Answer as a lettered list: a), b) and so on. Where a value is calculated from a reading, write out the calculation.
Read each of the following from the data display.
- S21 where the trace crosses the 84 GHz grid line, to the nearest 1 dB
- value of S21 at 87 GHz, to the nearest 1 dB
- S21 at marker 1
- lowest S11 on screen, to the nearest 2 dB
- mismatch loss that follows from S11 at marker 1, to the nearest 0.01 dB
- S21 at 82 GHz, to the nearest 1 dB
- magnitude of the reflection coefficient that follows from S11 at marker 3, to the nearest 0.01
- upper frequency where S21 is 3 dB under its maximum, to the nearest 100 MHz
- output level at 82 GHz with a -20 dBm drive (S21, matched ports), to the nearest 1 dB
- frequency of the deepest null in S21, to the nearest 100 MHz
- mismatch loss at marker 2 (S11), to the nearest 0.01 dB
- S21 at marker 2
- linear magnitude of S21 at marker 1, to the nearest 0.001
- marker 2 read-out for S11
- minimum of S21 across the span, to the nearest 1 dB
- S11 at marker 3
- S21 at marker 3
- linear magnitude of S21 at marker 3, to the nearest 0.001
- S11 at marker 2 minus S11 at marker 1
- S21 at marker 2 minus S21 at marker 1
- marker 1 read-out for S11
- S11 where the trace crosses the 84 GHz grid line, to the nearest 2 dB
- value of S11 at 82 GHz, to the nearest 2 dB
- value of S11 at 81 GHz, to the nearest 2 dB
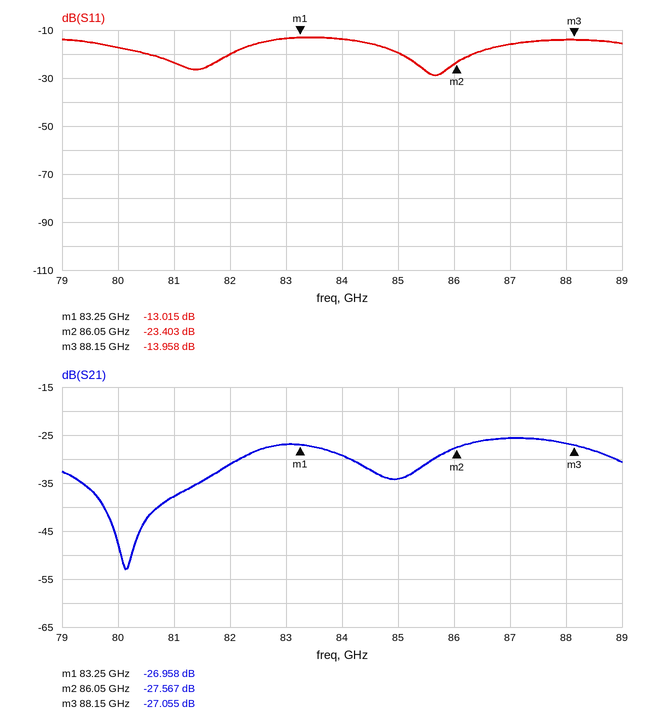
a) -29 dB
b) -26 dB
c) -26.958 dB
d) -28 dB
e) −10 log10(1 − 10^(-13.015/10)) ≈ 0.22 dB
f) -31 dB
g) 10^(-13.958/20) ≈ 0.20
h) 88.6 GHz
i) -20 dBm + (-31 dB) = -51 dBm
j) 80.1 GHz
k) −10 log10(1 − 10^(-23.403/10)) ≈ 0.02 dB
l) -27.567 dB
m) 10^(-26.958/20) ≈ 0.045
n) -23.403 dB
o) -53 dB
p) -13.958 dB
q) -27.055 dB
r) 10^(-27.055/20) ≈ 0.044
s) -23.403 − (-13.015) = -10.388 dB
t) -27.567 − (-26.958) = -0.609 dB
u) -13.015 dB
v) -14 dB
w) -20 dB
x) -24 dB
